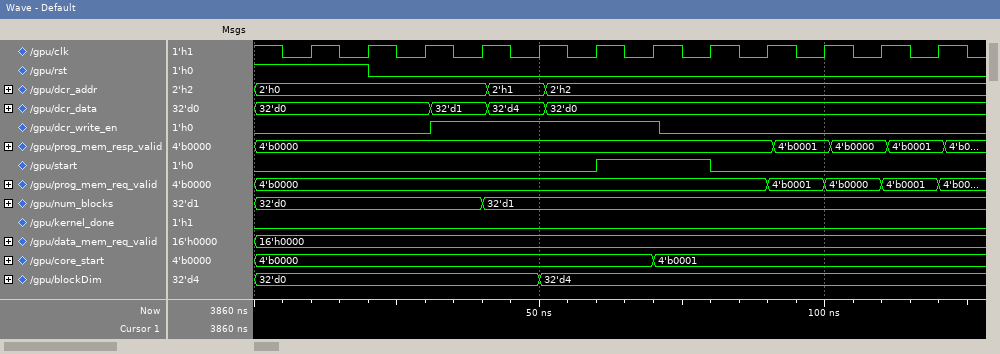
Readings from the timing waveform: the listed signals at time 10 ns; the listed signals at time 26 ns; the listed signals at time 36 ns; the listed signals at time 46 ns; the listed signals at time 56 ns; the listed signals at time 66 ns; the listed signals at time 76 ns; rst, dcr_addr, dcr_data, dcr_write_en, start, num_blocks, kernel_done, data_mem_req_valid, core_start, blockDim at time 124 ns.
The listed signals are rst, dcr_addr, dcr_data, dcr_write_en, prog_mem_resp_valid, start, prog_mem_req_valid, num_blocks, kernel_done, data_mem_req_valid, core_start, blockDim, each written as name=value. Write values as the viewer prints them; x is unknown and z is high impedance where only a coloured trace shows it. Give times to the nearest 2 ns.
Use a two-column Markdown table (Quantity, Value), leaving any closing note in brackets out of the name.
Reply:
| Quantity | Value |
|---|---|
| the listed signals at time 10 ns | rst=1, dcr_addr=2'h0, dcr_data=32'd0, dcr_write_en=0, prog_mem_resp_valid=4'b0000, start=0, prog_mem_req_valid=4'b0000, num_blocks=32'd0, kernel_done=0, data_mem_req_valid=16'h0000, core_start=4'b0000, blockDim=32'd0 |
| the listed signals at time 26 ns | rst=0, dcr_addr=2'h0, dcr_data=32'd0, dcr_write_en=0, prog_mem_resp_valid=4'b0000, start=0, prog_mem_req_valid=4'b0000, num_blocks=32'd0, kernel_done=0, data_mem_req_valid=16'h0000, core_start=4'b0000, blockDim=32'd0 |
| the listed signals at time 36 ns | rst=0, dcr_addr=2'h0, dcr_data=32'd1, dcr_write_en=1, prog_mem_resp_valid=4'b0000, start=0, prog_mem_req_valid=4'b0000, num_blocks=32'd0, kernel_done=0, data_mem_req_valid=16'h0000, core_start=4'b0000, blockDim=32'd0 |
| the listed signals at time 46 ns | rst=0, dcr_addr=2'h1, dcr_data=32'd4, dcr_write_en=1, prog_mem_resp_valid=4'b0000, start=0, prog_mem_req_valid=4'b0000, num_blocks=32'd1, kernel_done=0, data_mem_req_valid=16'h0000, core_start=4'b0000, blockDim=32'd0 |
| the listed signals at time 56 ns | rst=0, dcr_addr=2'h2, dcr_data=32'd0, dcr_write_en=1, prog_mem_resp_valid=4'b0000, start=0, prog_mem_req_valid=4'b0000, num_blocks=32'd1, kernel_done=0, data_mem_req_valid=16'h0000, core_start=4'b0000, blockDim=32'd4 |
| the listed signals at time 66 ns | rst=0, dcr_addr=2'h2, dcr_data=32'd0, dcr_write_en=1, prog_mem_resp_valid=4'b0000, start=1, prog_mem_req_valid=4'b0000, num_blocks=32'd1, kernel_done=0, data_mem_req_valid=16'h0000, core_start=4'b0000, blockDim=32'd4 |
| the listed signals at time 76 ns | rst=0, dcr_addr=2'h2, dcr_data=32'd0, dcr_write_en=0, prog_mem_resp_valid=4'b0000, start=1, prog_mem_req_valid=4'b0000, num_blocks=32'd1, kernel_done=0, data_mem_req_valid=16'h0000, core_start=4'b0001, blockDim=32'd4 |
| rst, dcr_addr, dcr_data, dcr_write_en, start, num_blocks, kernel_done, data_mem_req_valid, core_start, blockDim at time 124 ns | rst=0, dcr_addr=2'h2, dcr_data=32'd0, dcr_write_en=0, start=0, num_blocks=32'd1, kernel_done=0, data_mem_req_valid=16'h0000, core_start=4'b0001, blockDim=32'd4 |
